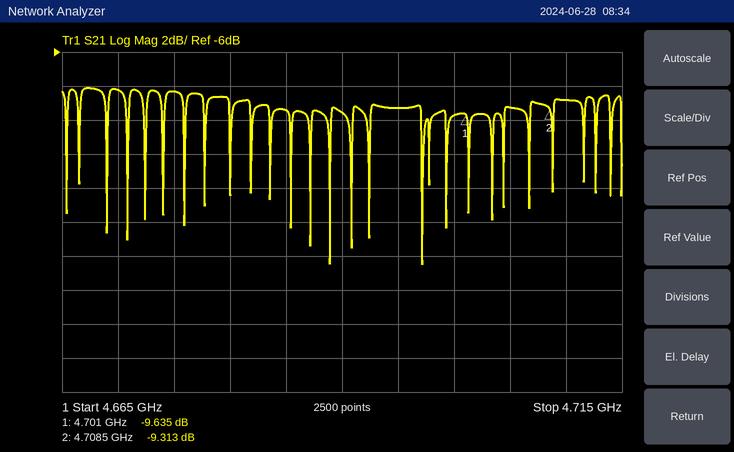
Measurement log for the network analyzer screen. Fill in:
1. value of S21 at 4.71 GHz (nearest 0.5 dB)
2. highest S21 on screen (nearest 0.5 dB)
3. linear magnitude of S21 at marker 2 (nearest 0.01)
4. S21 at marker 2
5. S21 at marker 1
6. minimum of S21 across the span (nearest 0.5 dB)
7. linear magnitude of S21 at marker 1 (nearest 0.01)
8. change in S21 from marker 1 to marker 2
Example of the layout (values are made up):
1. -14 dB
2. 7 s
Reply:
1. -9.0 dB
2. -8.0 dB
3. 0.34
4. -9.313 dB
5. -9.635 dB
6. -18.5 dB
7. 0.33
8. 0.322 dB
